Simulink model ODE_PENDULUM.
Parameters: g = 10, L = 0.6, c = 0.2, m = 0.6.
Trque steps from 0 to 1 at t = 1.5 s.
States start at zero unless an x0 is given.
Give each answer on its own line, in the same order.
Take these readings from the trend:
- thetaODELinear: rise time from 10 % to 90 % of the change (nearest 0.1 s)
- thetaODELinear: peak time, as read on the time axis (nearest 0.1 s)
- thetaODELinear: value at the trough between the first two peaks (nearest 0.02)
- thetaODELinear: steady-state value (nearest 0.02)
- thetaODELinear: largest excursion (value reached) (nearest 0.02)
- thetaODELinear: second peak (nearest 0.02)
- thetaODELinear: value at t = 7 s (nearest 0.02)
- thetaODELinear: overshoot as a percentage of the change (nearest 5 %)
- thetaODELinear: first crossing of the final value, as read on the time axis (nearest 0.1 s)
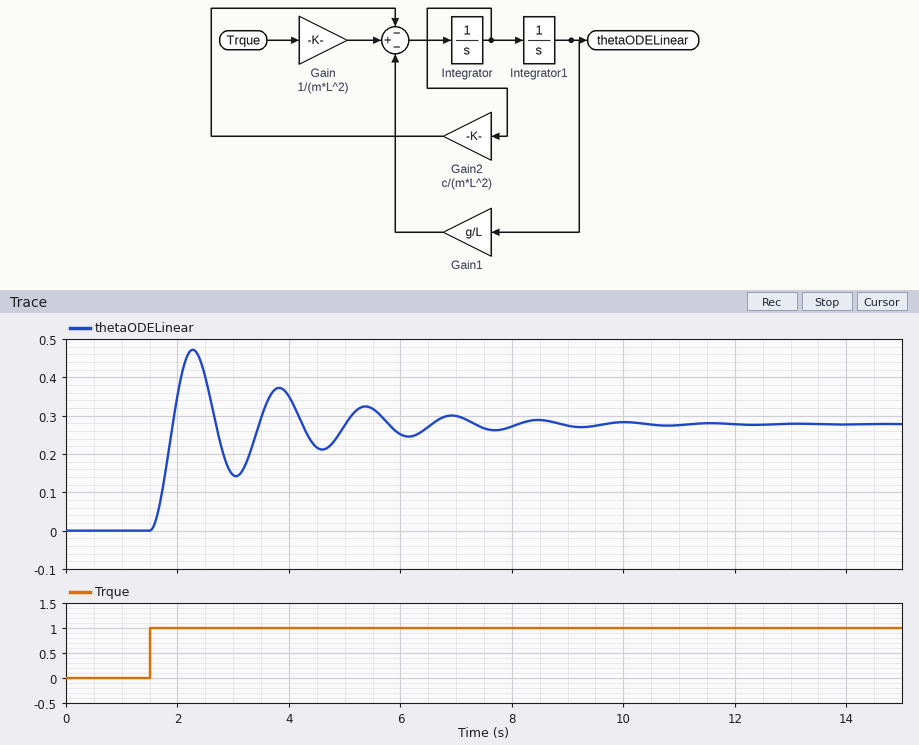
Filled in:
0.3 s
2.3 s
0.14
0.28
0.48
0.38
0.30
70 %
1.9 s
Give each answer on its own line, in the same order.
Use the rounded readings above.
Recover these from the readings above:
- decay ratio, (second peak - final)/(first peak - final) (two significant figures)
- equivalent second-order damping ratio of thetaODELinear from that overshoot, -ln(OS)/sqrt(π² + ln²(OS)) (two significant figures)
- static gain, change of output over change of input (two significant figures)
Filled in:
0.50
0.11
0.28
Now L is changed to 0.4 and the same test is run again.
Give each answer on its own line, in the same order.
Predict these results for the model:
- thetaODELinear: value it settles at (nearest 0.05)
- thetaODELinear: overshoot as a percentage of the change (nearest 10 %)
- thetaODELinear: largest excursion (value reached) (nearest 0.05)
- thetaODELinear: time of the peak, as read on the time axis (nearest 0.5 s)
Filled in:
0.40
50 %
0.65
2.0 s
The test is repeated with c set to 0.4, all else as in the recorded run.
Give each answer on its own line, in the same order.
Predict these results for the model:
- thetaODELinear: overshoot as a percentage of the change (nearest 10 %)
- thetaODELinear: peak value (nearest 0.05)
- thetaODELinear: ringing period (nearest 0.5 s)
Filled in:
50 %
0.40
1.5 s
